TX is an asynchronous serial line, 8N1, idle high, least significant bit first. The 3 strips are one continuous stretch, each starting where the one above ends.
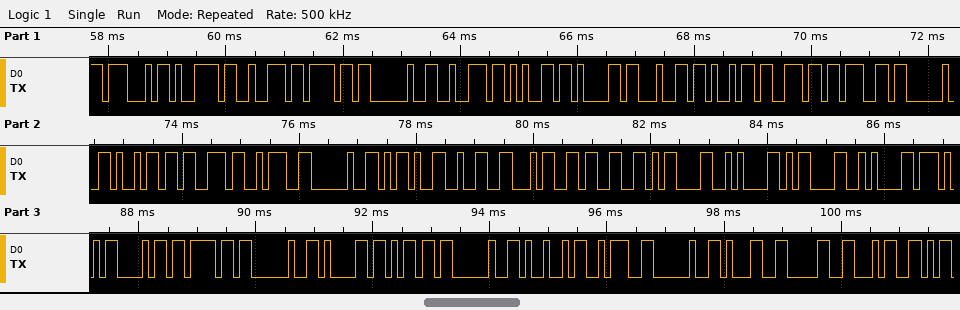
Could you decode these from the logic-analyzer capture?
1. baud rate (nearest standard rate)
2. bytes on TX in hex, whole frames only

9600 baud
47 79 72 6F 20 72 65 61 64 69 6E 67 20 69 73 3A 20 2D 32 34 33 0D 0A 0D 0A 57 68 6F 20 61 6D 20 49 3A 20 31 30 34
